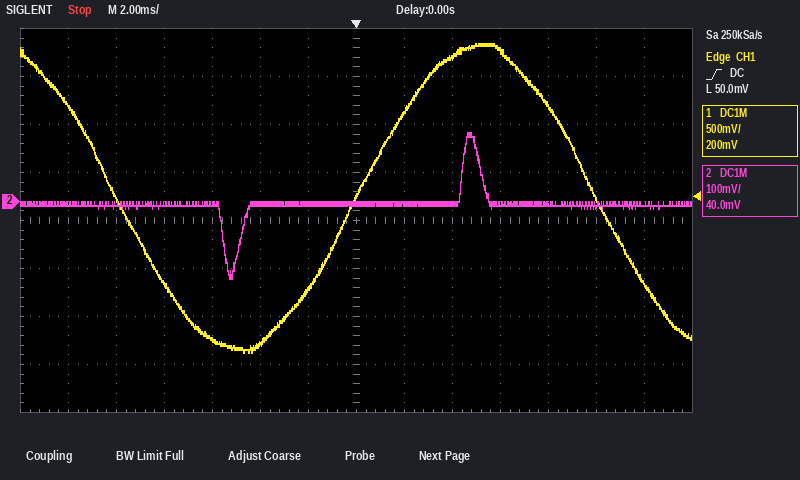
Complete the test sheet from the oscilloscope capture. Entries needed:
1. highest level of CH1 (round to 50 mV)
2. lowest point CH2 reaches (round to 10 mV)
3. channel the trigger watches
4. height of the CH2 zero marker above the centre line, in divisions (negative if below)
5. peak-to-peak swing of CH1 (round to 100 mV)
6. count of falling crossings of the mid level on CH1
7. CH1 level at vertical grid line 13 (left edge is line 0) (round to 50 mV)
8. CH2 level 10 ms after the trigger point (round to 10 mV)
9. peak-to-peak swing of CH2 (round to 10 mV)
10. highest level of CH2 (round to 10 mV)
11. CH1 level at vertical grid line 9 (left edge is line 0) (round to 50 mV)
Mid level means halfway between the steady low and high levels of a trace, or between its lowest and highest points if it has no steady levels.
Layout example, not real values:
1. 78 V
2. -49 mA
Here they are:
1. 1.65 V
2. -160 mV
3. CH1
4. +0.4 div
5. 3.20 V
6. 2
7. -850 mV
8. -10 mV
9. 300 mV
10. 140 mV
11. 1.50 V
